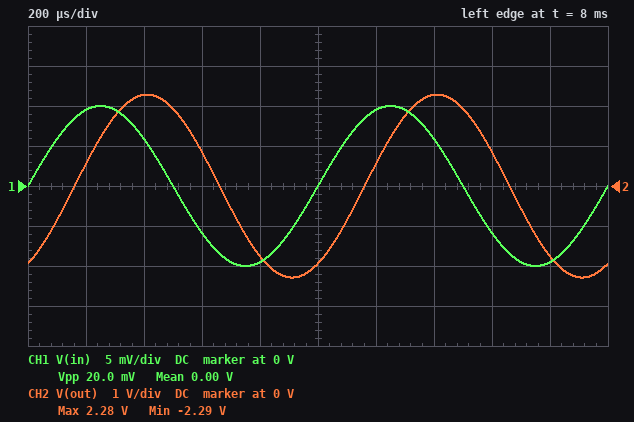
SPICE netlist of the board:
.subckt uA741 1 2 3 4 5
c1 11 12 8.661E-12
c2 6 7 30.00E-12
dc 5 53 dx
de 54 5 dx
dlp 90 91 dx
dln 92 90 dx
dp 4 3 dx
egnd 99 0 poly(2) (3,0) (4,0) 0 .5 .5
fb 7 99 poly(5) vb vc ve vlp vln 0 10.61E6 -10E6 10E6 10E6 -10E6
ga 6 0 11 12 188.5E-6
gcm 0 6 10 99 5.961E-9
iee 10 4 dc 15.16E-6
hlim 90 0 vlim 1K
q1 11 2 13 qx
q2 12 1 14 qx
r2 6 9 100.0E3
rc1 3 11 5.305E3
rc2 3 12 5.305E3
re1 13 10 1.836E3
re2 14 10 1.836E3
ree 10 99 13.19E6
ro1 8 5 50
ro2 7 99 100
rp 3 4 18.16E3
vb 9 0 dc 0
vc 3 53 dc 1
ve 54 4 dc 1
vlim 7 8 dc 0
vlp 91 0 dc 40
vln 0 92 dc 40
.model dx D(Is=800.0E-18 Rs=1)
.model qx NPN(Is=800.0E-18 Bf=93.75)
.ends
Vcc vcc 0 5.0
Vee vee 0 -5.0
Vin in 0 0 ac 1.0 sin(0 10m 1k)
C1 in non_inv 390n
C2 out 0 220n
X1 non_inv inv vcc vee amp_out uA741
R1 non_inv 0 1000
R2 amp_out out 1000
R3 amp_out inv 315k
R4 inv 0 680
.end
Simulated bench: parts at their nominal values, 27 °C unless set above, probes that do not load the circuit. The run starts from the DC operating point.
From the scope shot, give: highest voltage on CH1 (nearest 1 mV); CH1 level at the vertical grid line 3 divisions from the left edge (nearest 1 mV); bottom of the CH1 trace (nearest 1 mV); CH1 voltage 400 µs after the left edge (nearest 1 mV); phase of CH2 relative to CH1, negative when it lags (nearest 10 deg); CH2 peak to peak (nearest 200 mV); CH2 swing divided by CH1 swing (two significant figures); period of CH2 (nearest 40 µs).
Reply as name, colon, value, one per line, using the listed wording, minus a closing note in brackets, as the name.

highest voltage on CH1: 10 mV
CH1 level at the vertical grid line 3 divisions from the left edge: -6 mV
bottom of the CH1 trace: -10 mV
CH1 voltage 400 µs after the left edge: 6 mV
phase of CH2 relative to CH1, negative when it lags: -60 deg
CH2 peak to peak: 4.6 V
CH2 swing divided by CH1 swing: 230
period of CH2: 1.00 ms
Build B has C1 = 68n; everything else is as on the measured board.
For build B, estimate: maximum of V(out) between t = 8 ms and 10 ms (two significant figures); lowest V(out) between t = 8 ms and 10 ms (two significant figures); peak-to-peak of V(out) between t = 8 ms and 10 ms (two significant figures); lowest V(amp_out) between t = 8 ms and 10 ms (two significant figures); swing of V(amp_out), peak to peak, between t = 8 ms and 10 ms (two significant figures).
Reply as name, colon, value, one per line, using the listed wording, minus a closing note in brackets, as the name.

maximum of V(out) between t = 8 ms and 10 ms: 970 mV
lowest V(out) between t = 8 ms and 10 ms: -970 mV
peak-to-peak of V(out) between t = 8 ms and 10 ms: 1.9 V
lowest V(amp_out) between t = 8 ms and 10 ms: -1.7 V
swing of V(amp_out), peak to peak, between t = 8 ms and 10 ms: 3.3 V
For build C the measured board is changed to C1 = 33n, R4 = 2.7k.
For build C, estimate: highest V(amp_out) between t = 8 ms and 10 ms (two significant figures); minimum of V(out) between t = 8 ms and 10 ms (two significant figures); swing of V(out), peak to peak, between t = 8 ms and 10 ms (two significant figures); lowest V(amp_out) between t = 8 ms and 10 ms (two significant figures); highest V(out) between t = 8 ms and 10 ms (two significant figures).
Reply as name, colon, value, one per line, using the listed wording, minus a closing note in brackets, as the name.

highest V(amp_out) between t = 8 ms and 10 ms: 260 mV
minimum of V(out) between t = 8 ms and 10 ms: -120 mV
swing of V(out), peak to peak, between t = 8 ms and 10 ms: 280 mV
lowest V(amp_out) between t = 8 ms and 10 ms: -220 mV
highest V(out) between t = 8 ms and 10 ms: 160 mV
